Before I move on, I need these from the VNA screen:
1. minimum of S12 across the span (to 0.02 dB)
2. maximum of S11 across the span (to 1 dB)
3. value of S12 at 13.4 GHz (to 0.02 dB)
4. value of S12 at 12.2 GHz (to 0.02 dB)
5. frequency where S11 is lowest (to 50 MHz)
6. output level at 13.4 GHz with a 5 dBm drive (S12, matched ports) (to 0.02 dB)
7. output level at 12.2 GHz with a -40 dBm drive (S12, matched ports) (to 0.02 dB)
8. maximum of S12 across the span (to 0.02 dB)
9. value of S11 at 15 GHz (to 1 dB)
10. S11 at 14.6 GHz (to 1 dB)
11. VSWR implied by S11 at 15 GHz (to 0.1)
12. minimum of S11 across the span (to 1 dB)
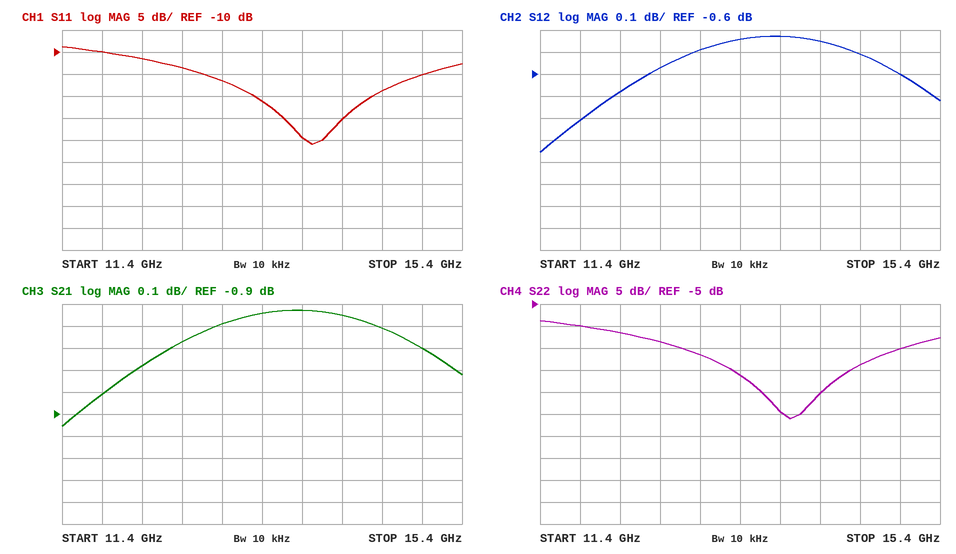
-0.96 dB
-9 dB
-0.44 dB
-0.68 dB
13.90 GHz
4.56 dBm
-40.68 dBm
-0.42 dB
-15 dB
-19 dB
1.4
-31 dB
